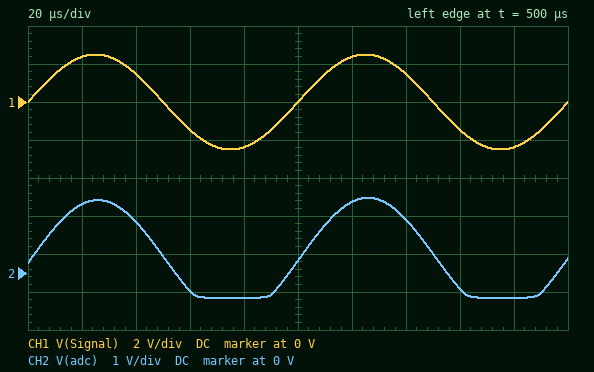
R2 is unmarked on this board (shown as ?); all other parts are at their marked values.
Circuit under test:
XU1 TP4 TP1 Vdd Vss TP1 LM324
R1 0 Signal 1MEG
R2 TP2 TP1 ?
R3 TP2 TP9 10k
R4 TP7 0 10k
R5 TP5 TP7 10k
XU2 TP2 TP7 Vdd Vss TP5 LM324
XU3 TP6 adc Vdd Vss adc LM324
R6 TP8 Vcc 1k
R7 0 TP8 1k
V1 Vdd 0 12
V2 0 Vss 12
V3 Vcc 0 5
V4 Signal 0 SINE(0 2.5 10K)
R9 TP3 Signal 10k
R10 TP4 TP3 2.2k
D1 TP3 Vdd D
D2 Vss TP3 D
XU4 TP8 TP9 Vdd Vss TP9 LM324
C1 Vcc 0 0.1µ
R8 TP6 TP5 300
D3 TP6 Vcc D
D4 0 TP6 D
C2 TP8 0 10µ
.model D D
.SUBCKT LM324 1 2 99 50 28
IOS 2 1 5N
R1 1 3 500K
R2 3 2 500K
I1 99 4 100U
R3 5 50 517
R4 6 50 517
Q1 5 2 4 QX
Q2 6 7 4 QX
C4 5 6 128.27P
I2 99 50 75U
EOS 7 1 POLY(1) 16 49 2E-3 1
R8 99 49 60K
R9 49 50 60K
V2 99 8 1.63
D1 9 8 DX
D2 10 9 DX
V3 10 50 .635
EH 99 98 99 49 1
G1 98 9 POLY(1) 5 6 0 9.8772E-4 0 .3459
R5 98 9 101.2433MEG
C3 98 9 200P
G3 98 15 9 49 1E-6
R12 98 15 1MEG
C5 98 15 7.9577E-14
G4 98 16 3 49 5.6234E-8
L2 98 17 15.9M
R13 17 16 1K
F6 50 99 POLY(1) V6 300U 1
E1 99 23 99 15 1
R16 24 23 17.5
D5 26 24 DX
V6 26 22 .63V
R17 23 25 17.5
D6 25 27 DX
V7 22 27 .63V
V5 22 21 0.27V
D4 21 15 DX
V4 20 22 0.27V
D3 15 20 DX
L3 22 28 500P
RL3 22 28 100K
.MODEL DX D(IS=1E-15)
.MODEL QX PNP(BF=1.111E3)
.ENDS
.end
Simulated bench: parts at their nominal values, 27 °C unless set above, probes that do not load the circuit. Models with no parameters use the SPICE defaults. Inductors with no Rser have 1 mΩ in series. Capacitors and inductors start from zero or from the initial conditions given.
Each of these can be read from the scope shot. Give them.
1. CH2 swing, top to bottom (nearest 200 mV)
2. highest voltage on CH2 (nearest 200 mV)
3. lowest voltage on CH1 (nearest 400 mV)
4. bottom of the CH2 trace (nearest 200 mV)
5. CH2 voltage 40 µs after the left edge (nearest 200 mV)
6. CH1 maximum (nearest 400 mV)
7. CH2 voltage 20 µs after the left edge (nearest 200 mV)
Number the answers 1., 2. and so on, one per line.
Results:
1. 2.6 V
2. 2.0 V
3. -2.4 V
4. -600 mV
5. 1.4 V
6. 2.4 V
7. 1.8 V
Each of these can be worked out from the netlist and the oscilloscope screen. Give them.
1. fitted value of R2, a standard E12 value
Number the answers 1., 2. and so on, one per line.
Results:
1. 22 kΩ
